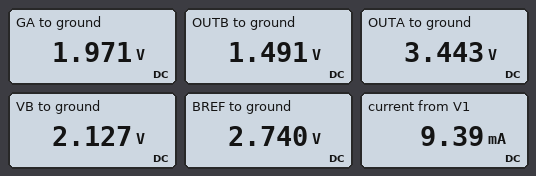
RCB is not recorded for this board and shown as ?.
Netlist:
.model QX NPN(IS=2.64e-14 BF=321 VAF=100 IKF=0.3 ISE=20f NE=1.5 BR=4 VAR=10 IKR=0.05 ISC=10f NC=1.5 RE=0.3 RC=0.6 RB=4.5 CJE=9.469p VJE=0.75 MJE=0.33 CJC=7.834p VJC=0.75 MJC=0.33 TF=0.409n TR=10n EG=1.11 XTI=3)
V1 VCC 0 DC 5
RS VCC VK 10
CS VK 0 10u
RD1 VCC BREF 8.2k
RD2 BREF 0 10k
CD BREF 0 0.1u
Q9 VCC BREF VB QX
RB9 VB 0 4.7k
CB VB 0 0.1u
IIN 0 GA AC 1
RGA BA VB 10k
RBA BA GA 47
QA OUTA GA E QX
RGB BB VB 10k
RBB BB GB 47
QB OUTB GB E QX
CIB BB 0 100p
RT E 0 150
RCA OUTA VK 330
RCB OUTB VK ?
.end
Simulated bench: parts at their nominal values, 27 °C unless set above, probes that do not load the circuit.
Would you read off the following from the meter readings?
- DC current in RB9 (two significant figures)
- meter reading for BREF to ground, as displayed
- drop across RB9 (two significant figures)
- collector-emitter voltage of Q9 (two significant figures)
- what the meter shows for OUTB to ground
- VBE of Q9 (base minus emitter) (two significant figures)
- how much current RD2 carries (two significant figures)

450 µA
2.740 V
2.1 V
2.9 V
1.491 V
610 mV
270 µA
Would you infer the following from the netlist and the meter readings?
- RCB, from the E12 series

820 Ω
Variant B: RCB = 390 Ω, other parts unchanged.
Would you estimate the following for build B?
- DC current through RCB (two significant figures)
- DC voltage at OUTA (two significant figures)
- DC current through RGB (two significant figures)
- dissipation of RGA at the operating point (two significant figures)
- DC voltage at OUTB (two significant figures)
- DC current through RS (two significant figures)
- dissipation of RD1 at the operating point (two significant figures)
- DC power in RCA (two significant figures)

4.3 mA
3.5 V
15 µA
2.3 µW
3.2 V
8.7 mA
620 µW
6.2 mW
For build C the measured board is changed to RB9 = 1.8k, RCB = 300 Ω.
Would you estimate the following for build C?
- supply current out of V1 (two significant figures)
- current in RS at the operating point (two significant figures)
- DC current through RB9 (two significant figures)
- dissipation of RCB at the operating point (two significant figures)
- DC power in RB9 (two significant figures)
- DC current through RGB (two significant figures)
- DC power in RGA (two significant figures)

9.9 mA
8.5 mA
1.2 mA
5.4 mW
2.4 mW
15 µA
2.2 µW
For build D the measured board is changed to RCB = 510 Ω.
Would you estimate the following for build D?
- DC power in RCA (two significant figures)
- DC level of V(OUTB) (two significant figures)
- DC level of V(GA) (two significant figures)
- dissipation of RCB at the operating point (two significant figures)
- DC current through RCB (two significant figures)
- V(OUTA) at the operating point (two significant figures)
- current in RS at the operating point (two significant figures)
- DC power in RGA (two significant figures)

6.2 mW
2.7 V
2.0 V
9.5 mW
4.3 mA
3.5 V
8.7 mA
2.3 µW
